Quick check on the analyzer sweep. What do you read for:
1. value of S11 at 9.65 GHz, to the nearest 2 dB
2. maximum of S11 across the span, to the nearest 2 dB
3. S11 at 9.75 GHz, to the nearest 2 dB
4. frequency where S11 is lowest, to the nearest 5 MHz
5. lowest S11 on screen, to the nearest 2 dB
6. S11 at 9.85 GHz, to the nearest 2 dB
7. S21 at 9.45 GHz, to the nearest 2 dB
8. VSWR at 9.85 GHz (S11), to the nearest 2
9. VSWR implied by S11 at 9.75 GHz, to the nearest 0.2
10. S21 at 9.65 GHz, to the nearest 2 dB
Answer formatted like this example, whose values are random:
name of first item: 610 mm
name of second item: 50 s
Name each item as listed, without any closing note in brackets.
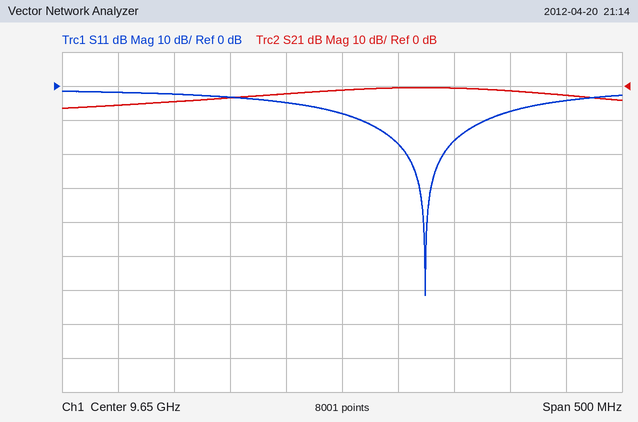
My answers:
value of S11 at 9.65 GHz, to the nearest 2 dB: -8 dB
maximum of S11 across the span, to the nearest 2 dB: -2 dB
S11 at 9.75 GHz, to the nearest 2 dB: -16 dB
frequency where S11 is lowest, to the nearest 5 MHz: 9.725 GHz
lowest S11 on screen, to the nearest 2 dB: -62 dB
S11 at 9.85 GHz, to the nearest 2 dB: -4 dB
S21 at 9.45 GHz, to the nearest 2 dB: -6 dB
VSWR at 9.85 GHz (S11), to the nearest 2: 4
VSWR implied by S11 at 9.75 GHz, to the nearest 0.2: 1.4
S21 at 9.65 GHz, to the nearest 2 dB: -2 dB
